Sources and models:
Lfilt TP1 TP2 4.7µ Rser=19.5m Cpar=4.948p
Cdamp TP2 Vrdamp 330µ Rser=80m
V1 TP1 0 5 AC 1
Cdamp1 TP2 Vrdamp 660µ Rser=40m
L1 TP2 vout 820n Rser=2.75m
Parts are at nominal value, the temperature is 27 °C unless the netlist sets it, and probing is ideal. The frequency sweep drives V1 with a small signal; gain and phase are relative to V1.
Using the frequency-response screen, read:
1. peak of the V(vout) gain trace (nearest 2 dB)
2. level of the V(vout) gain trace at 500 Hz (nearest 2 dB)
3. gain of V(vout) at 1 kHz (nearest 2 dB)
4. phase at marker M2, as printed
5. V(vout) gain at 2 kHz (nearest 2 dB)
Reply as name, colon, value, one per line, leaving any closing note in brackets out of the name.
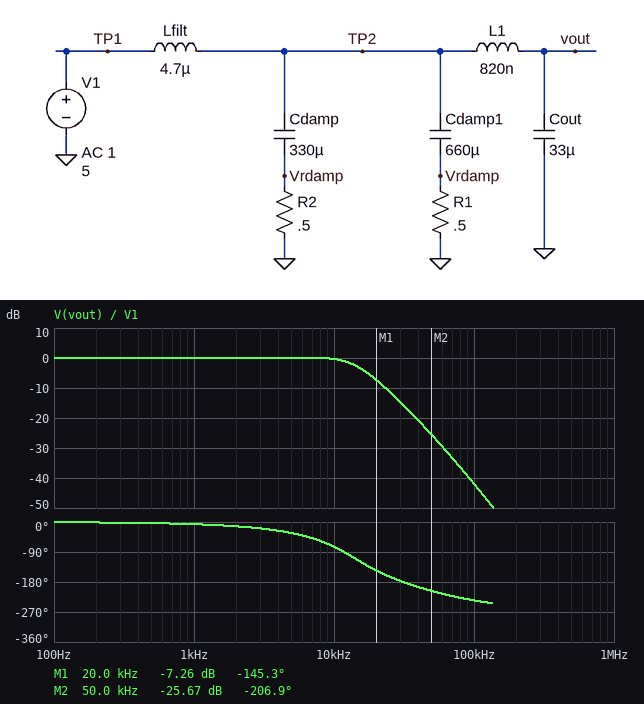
peak of the V(vout) gain trace: 0 dB
level of the V(vout) gain trace at 500 Hz: 0 dB
gain of V(vout) at 1 kHz: 0 dB
phase at marker M2, as printed: -206.9 deg
V(vout) gain at 2 kHz: 0 dB
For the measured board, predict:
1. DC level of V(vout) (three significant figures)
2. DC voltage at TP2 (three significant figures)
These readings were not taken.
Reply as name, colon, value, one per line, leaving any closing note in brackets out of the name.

DC level of V(vout): 5.00 V
DC voltage at TP2: 5.00 V
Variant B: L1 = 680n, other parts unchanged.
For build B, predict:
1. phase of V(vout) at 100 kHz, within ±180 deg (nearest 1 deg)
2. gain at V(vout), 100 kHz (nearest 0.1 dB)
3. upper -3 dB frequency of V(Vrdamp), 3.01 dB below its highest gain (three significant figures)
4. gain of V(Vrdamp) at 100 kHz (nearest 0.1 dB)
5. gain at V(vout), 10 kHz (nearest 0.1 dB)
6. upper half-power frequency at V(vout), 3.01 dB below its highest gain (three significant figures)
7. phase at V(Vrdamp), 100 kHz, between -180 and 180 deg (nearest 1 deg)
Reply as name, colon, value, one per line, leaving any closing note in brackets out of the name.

phase of V(vout) at 100 kHz, within ±180 deg: 130 deg
gain at V(vout), 100 kHz: -40.7 dB
upper -3 dB frequency of V(Vrdamp), 3.01 dB below its highest gain: 12.8 kHz
gain of V(Vrdamp) at 100 kHz: -23.7 dB
gain at V(vout), 10 kHz: -0.5 dB
upper half-power frequency at V(vout), 3.01 dB below its highest gain: 14.5 kHz
phase at V(Vrdamp), 100 kHz, between -180 and 180 deg: -50 deg
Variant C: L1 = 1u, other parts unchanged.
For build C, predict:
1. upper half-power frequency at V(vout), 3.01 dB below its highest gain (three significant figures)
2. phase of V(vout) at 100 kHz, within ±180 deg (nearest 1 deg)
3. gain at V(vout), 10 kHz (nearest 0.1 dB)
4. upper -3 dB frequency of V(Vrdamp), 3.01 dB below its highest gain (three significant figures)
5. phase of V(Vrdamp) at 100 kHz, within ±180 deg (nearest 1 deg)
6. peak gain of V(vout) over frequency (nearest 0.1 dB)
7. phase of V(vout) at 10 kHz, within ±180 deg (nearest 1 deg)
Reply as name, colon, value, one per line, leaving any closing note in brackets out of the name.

upper half-power frequency at V(vout), 3.01 dB below its highest gain: 15.0 kHz
phase of V(vout) at 100 kHz, within ±180 deg: 120 deg
gain at V(vout), 10 kHz: -0.1 dB
upper -3 dB frequency of V(Vrdamp), 3.01 dB below its highest gain: 12.6 kHz
phase of V(Vrdamp) at 100 kHz, within ±180 deg: -60 deg
peak gain of V(vout) over frequency: 0.2 dB
phase of V(vout) at 10 kHz, within ±180 deg: -75 deg
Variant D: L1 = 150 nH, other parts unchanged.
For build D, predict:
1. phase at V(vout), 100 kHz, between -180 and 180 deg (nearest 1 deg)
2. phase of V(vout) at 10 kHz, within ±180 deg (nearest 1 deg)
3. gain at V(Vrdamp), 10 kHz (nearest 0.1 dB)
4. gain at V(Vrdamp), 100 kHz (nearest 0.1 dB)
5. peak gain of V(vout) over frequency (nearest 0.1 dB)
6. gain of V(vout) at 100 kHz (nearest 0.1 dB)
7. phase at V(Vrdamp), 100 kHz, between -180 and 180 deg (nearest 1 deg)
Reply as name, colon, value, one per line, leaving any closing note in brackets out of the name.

phase at V(vout), 100 kHz, between -180 and 180 deg: 171 deg
phase of V(vout) at 10 kHz, within ±180 deg: -71 deg
gain at V(Vrdamp), 10 kHz: -2.3 dB
gain at V(Vrdamp), 100 kHz: -37.3 dB
peak gain of V(vout) over frequency: 0 dB
gain of V(vout) at 100 kHz: -36.1 dB
phase at V(Vrdamp), 100 kHz, between -180 and 180 deg: -12 deg
